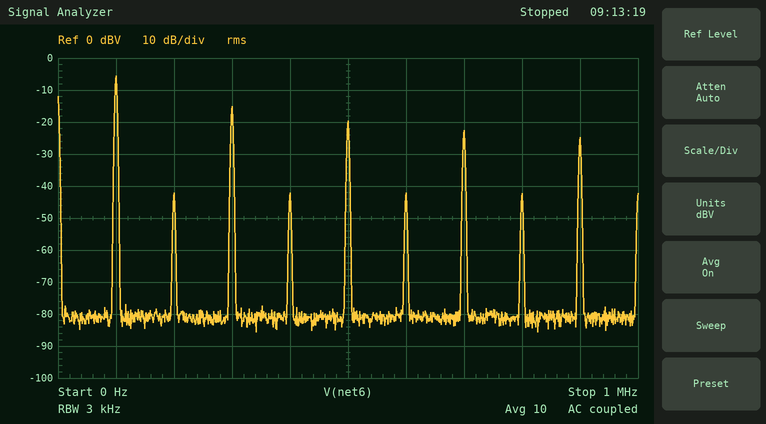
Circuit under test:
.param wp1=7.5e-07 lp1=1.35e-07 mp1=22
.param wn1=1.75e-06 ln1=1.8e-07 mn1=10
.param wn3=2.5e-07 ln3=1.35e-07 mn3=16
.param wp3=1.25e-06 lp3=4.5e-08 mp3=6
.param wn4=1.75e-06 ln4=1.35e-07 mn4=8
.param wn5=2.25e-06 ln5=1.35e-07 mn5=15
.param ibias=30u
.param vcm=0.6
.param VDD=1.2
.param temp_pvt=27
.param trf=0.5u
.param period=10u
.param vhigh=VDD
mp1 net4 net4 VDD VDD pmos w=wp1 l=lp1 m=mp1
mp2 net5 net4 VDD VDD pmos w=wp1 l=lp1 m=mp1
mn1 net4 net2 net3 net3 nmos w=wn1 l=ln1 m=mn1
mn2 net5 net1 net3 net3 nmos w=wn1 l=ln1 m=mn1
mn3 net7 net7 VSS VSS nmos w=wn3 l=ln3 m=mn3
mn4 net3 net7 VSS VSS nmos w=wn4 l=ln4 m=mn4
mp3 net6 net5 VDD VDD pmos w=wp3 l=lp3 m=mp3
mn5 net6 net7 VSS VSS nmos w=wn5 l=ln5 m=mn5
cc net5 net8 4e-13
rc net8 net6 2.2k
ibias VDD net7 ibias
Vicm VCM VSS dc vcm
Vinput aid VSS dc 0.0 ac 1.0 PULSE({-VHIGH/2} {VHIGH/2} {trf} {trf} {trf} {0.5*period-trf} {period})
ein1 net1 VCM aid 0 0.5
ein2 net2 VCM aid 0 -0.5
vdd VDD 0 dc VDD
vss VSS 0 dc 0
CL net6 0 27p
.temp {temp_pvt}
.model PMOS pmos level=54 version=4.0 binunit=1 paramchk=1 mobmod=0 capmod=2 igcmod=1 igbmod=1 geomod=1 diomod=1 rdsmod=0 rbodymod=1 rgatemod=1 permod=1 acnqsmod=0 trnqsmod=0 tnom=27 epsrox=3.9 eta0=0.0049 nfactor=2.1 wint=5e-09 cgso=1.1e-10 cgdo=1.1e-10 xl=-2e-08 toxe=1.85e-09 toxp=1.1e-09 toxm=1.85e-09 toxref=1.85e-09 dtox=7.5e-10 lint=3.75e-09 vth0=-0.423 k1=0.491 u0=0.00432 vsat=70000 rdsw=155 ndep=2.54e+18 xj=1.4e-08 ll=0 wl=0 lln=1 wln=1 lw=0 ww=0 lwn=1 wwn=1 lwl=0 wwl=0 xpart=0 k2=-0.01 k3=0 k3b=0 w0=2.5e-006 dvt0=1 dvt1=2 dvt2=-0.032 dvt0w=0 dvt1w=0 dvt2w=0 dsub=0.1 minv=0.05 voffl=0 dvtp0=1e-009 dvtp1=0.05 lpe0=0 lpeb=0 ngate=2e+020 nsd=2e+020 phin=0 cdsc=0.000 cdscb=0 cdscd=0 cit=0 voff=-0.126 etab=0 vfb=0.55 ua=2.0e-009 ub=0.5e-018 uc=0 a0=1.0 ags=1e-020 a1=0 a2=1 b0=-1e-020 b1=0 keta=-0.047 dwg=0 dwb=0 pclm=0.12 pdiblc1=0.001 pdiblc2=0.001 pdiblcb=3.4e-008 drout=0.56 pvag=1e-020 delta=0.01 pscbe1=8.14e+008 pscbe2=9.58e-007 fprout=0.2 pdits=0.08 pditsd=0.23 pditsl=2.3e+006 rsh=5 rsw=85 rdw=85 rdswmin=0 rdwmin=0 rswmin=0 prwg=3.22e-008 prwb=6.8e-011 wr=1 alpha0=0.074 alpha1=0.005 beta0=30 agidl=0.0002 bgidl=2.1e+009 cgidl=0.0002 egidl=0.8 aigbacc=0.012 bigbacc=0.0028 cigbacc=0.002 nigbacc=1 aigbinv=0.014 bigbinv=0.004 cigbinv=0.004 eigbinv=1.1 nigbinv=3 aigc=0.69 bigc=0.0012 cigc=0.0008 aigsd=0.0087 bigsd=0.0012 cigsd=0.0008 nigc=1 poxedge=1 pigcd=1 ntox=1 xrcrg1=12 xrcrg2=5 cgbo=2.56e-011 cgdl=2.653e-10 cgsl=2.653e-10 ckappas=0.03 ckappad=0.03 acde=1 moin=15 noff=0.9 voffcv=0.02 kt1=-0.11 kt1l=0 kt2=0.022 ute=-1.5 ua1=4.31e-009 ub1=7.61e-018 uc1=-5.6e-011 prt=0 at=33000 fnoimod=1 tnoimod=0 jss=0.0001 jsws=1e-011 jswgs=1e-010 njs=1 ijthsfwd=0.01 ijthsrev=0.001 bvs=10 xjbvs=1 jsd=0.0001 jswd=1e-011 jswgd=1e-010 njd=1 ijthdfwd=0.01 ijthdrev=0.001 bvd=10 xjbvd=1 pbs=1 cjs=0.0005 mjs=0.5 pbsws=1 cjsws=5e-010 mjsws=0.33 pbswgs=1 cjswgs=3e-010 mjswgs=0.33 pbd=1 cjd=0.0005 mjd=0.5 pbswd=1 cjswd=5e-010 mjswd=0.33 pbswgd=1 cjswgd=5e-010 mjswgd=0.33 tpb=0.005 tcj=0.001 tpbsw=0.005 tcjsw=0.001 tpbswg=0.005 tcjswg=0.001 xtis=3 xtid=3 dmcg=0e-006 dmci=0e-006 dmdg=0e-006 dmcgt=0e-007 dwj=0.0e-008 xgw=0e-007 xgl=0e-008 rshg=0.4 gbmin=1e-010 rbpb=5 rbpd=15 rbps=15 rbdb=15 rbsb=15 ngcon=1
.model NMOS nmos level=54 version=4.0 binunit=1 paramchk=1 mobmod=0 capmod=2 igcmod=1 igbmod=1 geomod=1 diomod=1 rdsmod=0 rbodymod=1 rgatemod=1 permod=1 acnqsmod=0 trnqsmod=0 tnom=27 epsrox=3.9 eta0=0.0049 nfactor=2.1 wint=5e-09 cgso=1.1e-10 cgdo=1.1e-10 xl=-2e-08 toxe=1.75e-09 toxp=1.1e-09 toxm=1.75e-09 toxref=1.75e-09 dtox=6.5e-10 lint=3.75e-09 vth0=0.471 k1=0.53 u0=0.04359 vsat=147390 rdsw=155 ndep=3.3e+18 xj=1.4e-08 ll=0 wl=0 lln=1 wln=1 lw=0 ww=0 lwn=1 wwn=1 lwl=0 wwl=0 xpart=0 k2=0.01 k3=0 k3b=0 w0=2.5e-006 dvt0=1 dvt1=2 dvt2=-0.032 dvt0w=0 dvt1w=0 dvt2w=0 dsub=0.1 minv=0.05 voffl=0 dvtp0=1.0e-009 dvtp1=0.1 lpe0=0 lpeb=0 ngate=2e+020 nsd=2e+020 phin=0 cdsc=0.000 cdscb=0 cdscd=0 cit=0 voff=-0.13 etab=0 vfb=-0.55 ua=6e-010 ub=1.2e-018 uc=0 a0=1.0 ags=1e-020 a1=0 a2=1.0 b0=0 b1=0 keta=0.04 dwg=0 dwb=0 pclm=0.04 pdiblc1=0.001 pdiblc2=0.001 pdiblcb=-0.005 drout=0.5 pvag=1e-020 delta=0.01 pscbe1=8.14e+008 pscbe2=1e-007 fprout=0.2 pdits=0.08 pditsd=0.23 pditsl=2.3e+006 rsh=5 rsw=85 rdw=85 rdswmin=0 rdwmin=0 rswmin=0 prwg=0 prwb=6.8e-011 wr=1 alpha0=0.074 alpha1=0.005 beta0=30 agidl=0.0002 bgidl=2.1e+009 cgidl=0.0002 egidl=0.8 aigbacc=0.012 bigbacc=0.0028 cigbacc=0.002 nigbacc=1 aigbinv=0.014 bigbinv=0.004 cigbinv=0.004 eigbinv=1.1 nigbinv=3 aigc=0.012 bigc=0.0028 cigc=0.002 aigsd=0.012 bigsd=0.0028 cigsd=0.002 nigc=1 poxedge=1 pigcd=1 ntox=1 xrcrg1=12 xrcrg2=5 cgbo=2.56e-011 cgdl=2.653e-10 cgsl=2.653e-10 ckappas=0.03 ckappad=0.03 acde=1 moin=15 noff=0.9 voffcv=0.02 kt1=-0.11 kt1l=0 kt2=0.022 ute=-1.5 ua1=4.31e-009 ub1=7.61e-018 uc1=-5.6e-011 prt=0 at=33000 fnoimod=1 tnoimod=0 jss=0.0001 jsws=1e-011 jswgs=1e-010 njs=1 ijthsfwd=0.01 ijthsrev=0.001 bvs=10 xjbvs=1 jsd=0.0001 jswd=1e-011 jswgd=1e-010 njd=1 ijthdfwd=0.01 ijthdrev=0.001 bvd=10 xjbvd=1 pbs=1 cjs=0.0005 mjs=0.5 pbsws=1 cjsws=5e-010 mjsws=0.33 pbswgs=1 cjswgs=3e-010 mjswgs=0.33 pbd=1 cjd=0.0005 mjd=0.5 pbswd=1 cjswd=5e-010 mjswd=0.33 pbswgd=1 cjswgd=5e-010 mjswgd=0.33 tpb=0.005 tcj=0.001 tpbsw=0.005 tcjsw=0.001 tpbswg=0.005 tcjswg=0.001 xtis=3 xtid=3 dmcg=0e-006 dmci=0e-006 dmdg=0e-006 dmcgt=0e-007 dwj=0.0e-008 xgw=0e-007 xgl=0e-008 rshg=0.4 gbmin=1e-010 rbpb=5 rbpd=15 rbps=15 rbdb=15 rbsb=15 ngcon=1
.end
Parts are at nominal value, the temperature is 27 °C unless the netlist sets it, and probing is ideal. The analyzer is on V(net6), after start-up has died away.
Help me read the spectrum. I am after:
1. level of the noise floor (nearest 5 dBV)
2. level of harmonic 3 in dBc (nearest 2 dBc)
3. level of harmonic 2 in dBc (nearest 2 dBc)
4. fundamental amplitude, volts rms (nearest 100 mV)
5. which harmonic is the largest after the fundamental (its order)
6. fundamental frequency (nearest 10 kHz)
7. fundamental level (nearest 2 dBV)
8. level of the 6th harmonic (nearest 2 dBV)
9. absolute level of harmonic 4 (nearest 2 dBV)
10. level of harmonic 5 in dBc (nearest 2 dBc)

-80 dBV
-10 dBc
-36 dBc
500 mV
3
100 kHz
-6 dBV
-42 dBV
-42 dBV
-14 dBc
